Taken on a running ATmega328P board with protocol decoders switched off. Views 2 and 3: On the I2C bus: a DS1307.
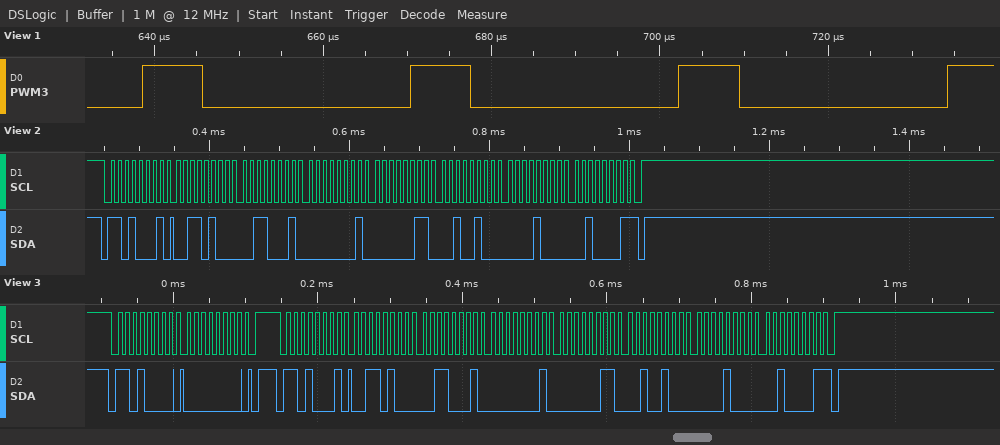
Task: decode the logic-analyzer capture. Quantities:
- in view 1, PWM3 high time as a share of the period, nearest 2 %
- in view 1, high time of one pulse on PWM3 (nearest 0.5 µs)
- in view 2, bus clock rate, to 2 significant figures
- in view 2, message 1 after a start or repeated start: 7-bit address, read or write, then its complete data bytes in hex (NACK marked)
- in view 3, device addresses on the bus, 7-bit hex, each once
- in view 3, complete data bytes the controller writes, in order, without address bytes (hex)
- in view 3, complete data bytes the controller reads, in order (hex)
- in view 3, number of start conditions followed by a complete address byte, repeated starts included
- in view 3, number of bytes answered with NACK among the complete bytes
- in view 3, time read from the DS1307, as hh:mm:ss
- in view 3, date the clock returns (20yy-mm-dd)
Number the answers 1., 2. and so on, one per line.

1. 22 %
2. 7.0 µs
3. 100 kHz
4. 0x68 read: 34 31 01 03 24 08 21 NACK
5. 0x68
6. 00
7. 34 31 01 03 24 08 21
8. 2
9. 1
10. 01:31:34
11. 2021-08-24
